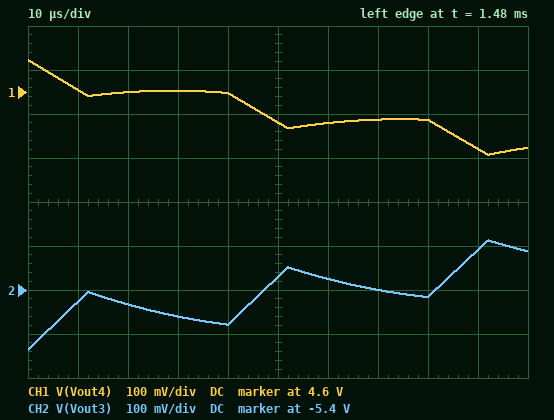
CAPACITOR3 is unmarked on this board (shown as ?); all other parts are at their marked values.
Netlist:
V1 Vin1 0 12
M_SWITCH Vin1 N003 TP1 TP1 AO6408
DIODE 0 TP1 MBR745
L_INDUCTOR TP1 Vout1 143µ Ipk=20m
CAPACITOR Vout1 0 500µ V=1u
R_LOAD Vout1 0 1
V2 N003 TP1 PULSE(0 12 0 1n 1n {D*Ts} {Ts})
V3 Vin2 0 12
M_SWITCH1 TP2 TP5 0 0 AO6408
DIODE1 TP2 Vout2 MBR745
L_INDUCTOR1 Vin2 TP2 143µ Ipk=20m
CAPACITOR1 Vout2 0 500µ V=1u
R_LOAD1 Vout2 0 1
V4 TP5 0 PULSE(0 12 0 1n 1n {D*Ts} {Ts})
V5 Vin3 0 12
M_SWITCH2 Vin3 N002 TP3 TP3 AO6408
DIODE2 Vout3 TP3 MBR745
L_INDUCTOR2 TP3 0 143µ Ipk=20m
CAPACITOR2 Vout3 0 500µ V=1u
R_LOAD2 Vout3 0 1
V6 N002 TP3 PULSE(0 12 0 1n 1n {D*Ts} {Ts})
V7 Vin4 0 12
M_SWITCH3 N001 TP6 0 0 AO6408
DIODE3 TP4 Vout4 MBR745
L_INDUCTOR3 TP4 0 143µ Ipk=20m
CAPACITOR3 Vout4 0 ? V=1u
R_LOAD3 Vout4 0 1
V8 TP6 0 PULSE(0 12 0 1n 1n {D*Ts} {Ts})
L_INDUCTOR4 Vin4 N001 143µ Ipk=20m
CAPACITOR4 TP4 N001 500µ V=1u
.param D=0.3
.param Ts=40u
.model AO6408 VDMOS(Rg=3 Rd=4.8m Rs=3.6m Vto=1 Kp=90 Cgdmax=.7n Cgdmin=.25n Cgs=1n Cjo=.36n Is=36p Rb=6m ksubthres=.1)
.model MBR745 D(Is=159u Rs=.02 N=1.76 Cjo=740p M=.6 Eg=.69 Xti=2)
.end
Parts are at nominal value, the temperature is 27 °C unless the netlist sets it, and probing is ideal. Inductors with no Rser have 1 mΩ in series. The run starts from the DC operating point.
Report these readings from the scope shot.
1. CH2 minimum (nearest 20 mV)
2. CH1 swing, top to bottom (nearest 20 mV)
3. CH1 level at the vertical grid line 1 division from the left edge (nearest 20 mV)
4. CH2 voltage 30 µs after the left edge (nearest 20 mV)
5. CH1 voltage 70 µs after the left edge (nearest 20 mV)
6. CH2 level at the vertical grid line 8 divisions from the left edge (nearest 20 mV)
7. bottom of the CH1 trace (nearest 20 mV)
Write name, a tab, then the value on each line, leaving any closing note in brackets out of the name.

CH2 minimum	-5.54 V
CH1 swing, top to bottom	220 mV
CH1 level at the vertical grid line 1 division from the left edge	4.60 V
CH2 voltage 30 µs after the left edge	-5.46 V
CH1 voltage 70 µs after the left edge	4.54 V
CH2 level at the vertical grid line 8 divisions from the left edge	-5.42 V
bottom of the CH1 trace	4.46 V
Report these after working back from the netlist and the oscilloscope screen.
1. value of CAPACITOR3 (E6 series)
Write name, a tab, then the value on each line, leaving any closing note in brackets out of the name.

value of CAPACITOR3	680 µF
